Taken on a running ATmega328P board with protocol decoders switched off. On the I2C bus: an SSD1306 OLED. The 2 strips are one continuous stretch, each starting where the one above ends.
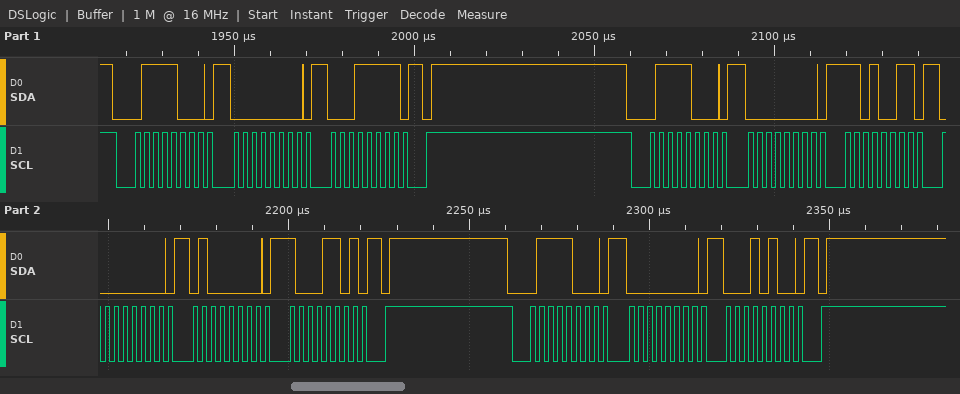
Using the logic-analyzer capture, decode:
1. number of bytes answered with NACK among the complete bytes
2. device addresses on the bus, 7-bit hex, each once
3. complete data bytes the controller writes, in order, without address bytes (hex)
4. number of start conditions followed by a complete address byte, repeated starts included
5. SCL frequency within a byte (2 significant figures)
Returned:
0
0x3C
00 1F 00 D3 00 40 8D 00 14
3
400 kHz
